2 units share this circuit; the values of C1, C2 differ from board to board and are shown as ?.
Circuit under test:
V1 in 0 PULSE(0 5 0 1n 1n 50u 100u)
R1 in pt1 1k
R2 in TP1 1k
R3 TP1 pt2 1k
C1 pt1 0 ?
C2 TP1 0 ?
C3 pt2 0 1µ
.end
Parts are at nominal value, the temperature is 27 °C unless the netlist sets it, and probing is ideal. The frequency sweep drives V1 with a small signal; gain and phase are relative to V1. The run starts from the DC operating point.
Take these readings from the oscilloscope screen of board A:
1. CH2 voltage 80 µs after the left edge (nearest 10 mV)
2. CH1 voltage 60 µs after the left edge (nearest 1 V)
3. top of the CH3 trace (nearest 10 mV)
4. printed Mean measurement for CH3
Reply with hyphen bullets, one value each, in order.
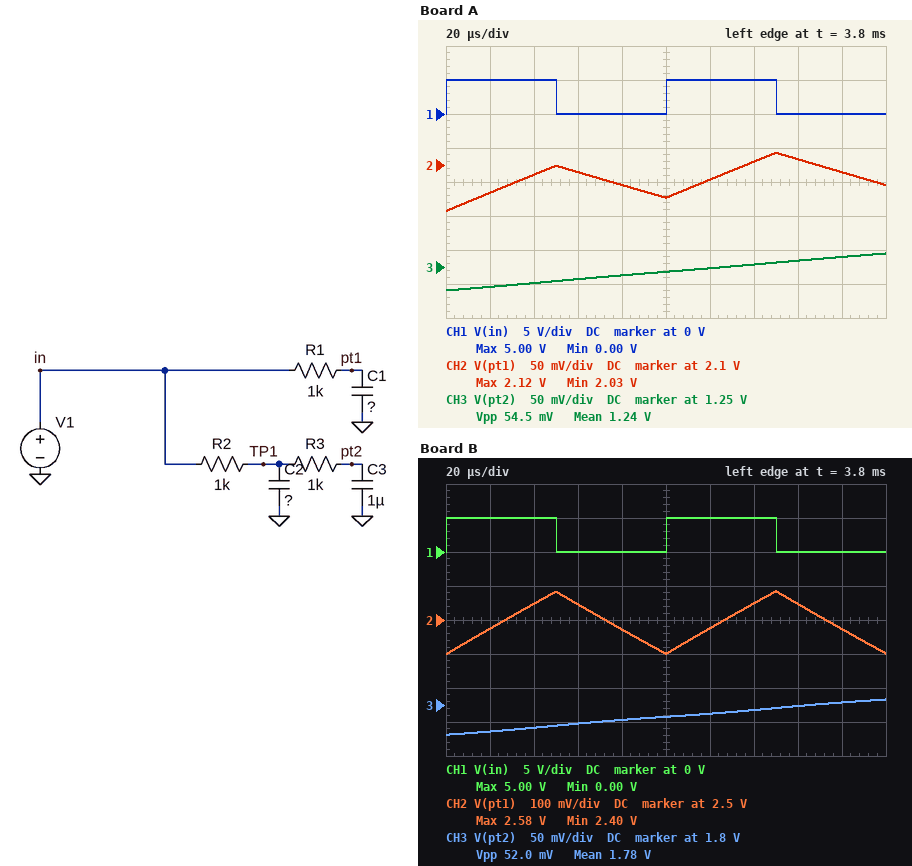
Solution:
- 2.07 V
- 0 V
- 1.27 V
- 1.24 V
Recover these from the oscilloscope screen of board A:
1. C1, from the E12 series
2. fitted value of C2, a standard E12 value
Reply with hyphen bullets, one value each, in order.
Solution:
- 2.2 µF
- 3.3 µF
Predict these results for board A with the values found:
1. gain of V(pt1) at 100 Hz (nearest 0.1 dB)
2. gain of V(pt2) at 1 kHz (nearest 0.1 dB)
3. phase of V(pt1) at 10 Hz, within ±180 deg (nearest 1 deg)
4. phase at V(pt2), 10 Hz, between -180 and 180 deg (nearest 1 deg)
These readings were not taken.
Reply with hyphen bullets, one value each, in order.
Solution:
- -4.6 dB
- -42.5 dB
- -8 deg
- -19 deg
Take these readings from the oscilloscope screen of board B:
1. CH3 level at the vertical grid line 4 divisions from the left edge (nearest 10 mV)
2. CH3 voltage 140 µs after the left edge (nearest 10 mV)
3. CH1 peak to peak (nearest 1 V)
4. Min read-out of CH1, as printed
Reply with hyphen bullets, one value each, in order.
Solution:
- 1.78 V
- 1.79 V
- 5 V
- 0.00 V
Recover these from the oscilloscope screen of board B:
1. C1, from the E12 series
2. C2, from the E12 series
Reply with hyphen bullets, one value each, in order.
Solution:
- 680 nF
- 1.2 µF
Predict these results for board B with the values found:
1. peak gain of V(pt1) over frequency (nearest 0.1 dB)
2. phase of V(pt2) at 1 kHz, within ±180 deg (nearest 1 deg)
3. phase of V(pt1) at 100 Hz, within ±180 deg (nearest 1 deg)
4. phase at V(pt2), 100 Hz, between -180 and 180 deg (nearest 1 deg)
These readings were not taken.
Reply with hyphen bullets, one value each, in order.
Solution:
- 0 dB
- -157 deg
- -23 deg
- -75 deg
